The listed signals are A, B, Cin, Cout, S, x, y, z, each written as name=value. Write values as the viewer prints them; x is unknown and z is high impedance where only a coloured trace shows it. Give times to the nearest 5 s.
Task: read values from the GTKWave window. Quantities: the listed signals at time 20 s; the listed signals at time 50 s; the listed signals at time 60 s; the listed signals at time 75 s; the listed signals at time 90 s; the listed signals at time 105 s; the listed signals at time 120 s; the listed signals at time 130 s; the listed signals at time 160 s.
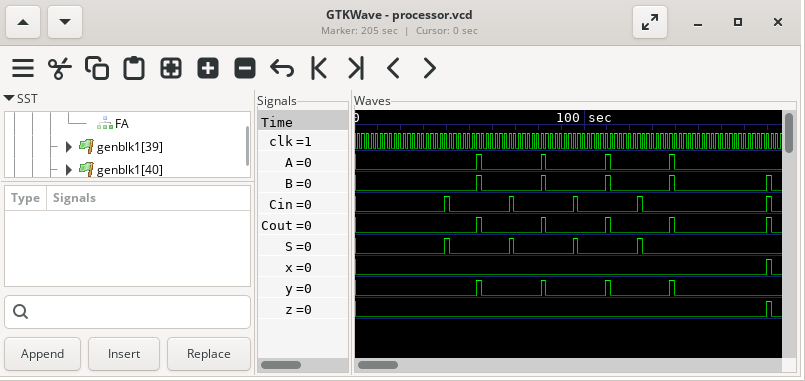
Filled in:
A=0, B=0, Cin=0, Cout=0, S=0, x=0, y=0, z=0
A=0, B=0, Cin=0, Cout=0, S=0, x=0, y=0, z=0
A=0, B=0, Cin=0, Cout=0, S=0, x=0, y=0, z=0
A=0, B=0, Cin=0, Cout=0, S=0, x=0, y=0, z=0
A=0, B=0, Cin=0, Cout=0, S=0, x=0, y=0, z=0
A=0, B=0, Cin=0, Cout=0, S=0, x=0, y=0, z=0
A=0, B=0, Cin=0, Cout=0, S=0, x=0, y=0, z=0
A=0, B=0, Cin=0, Cout=0, S=0, x=0, y=0, z=0
A=0, B=0, Cin=0, Cout=0, S=0, x=0, y=0, z=0
